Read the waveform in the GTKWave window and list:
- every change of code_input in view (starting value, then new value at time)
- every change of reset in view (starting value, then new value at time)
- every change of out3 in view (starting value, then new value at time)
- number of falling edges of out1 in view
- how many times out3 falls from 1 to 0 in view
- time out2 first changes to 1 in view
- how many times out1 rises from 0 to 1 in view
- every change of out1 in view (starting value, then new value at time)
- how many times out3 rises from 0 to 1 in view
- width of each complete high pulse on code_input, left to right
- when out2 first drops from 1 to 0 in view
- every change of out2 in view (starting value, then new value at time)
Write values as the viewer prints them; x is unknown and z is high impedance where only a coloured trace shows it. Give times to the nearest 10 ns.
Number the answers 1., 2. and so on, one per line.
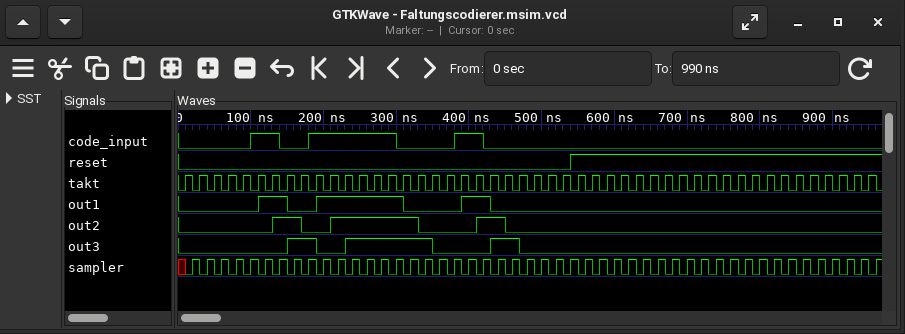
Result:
1. 0, 1 at 100 ns, 0 at 140 ns, 1 at 180 ns, 0 at 300 ns, 1 at 380 ns, 0 at 420 ns
2. 0, 1 at 540 ns
3. 0, 1 at 150 ns, 0 at 190 ns, 1 at 230 ns, 0 at 350 ns, 1 at 430 ns, 0 at 470 ns
4. 3
5. 3
6. 130 ns
7. 3
8. 0, 1 at 110 ns, 0 at 150 ns, 1 at 190 ns, 0 at 310 ns, 1 at 390 ns, 0 at 430 ns
9. 3
10. 40 ns, 120 ns, 40 ns
11. 170 ns
12. 0, 1 at 130 ns, 0 at 170 ns, 1 at 210 ns, 0 at 330 ns, 1 at 410 ns, 0 at 450 ns
